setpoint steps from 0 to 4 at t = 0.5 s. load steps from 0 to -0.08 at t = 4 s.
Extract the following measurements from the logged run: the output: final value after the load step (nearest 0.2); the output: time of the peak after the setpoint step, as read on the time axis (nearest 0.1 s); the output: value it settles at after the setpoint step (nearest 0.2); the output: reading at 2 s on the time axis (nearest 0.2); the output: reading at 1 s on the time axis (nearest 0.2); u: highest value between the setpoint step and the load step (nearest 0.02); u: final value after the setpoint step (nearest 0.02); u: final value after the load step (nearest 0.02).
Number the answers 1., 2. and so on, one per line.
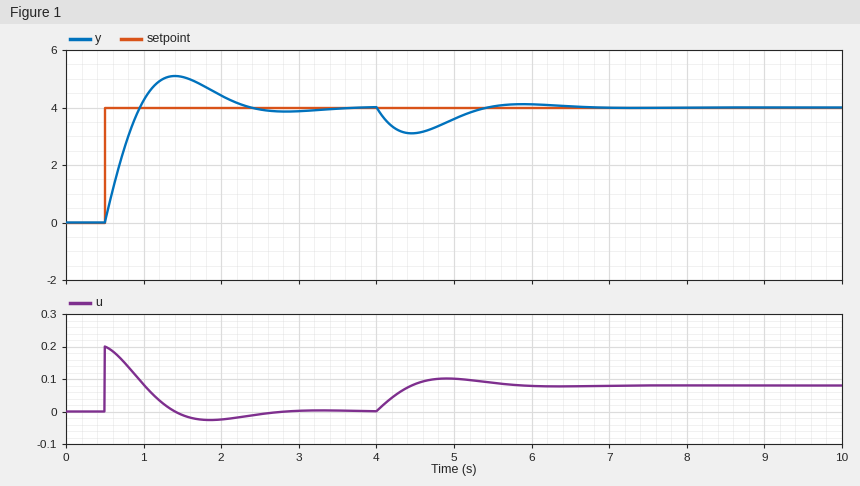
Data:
1. 4.0
2. 1.4 s
3. 4.0
4. 4.4
5. 4.2
6. 0.20
7. 0.00
8. 0.08
